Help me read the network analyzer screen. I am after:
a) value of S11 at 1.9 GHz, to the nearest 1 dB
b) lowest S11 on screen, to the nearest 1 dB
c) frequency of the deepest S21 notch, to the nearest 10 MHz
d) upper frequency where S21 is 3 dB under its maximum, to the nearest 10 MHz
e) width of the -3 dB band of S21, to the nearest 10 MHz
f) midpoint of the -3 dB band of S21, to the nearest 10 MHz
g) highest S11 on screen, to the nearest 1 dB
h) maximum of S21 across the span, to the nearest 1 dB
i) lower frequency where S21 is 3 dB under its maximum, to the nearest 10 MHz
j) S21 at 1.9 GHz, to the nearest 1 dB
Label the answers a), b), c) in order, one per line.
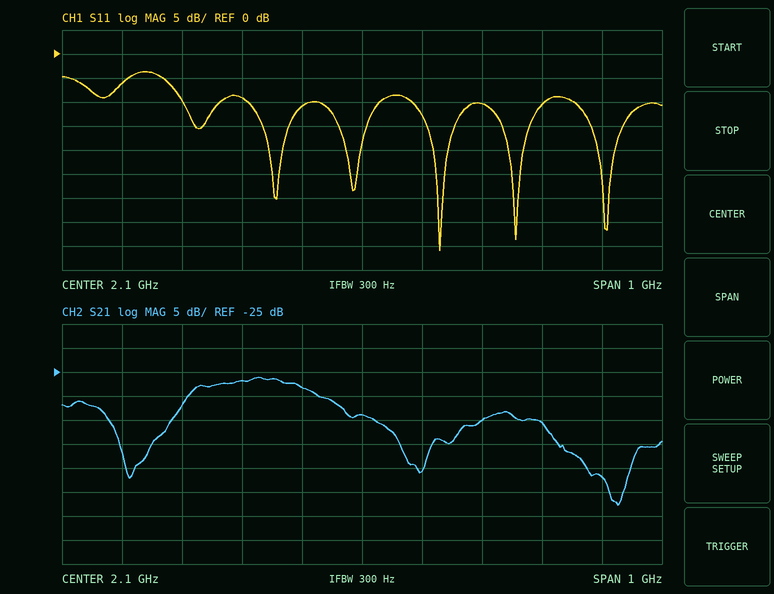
a) -9 dB
b) -41 dB
c) 2.53 GHz
d) 2.02 GHz
e) 200 MHz
f) 1.92 GHz
g) -4 dB
h) -26 dB
i) 1.82 GHz
j) -27 dB
